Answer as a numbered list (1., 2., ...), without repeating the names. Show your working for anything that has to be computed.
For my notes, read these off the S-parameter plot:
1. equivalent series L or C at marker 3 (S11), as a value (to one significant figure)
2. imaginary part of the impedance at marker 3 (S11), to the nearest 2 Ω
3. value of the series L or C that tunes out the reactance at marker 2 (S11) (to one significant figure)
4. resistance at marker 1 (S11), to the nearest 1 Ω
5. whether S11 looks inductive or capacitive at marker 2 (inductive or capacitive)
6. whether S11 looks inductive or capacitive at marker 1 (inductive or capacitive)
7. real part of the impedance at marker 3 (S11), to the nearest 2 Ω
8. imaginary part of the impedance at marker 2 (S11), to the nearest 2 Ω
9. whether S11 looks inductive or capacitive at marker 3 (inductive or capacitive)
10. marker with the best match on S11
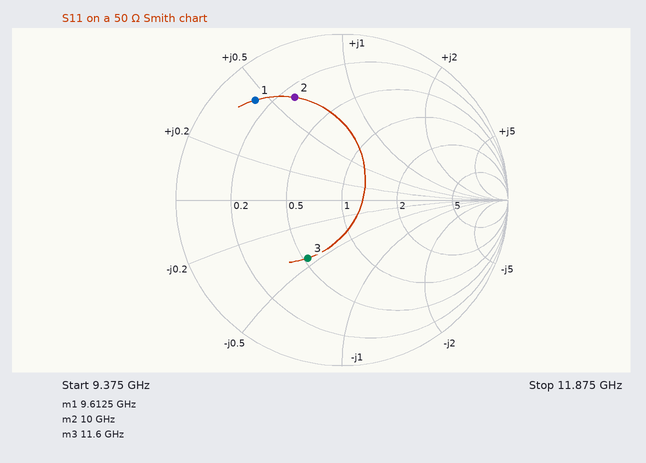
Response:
1. C = 1/(2π × 11.6 GHz × 22 Ω) ≈ 624 fF, so 600 fF to one significant figure
2. -22 Ω
3. C = 1/(2π × 10 GHz × 30 Ω) ≈ 531 fF, so 500 fF to one significant figure
4. 7 Ω
5. inductive
6. inductive
7. 26 Ω
8. +30 Ω
9. capacitive
10. marker 3
